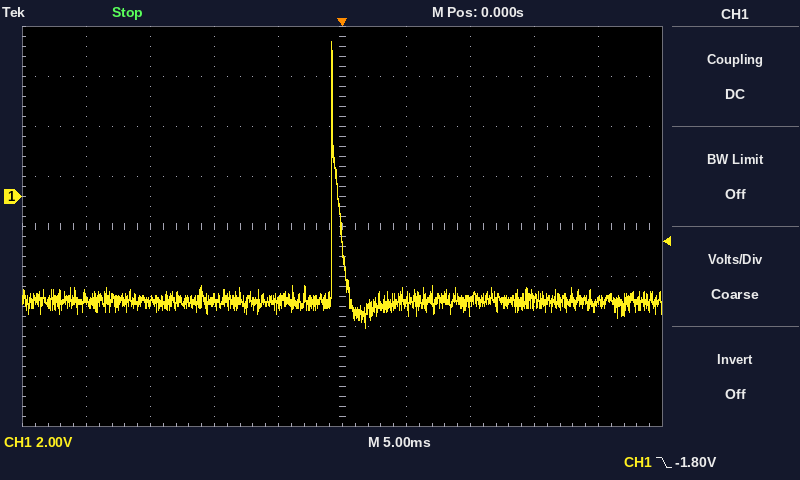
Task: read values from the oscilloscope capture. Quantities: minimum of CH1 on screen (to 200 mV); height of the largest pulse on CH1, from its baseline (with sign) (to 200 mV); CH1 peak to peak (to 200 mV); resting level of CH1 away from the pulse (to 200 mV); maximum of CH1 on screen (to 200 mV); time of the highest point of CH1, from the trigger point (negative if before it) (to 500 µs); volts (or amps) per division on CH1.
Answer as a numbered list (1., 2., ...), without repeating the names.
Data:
1. -5.2 V
2. +10.4 V
3. 11.4 V
4. -4.2 V
5. 6.2 V
6. -1.0 ms
7. 2 V
